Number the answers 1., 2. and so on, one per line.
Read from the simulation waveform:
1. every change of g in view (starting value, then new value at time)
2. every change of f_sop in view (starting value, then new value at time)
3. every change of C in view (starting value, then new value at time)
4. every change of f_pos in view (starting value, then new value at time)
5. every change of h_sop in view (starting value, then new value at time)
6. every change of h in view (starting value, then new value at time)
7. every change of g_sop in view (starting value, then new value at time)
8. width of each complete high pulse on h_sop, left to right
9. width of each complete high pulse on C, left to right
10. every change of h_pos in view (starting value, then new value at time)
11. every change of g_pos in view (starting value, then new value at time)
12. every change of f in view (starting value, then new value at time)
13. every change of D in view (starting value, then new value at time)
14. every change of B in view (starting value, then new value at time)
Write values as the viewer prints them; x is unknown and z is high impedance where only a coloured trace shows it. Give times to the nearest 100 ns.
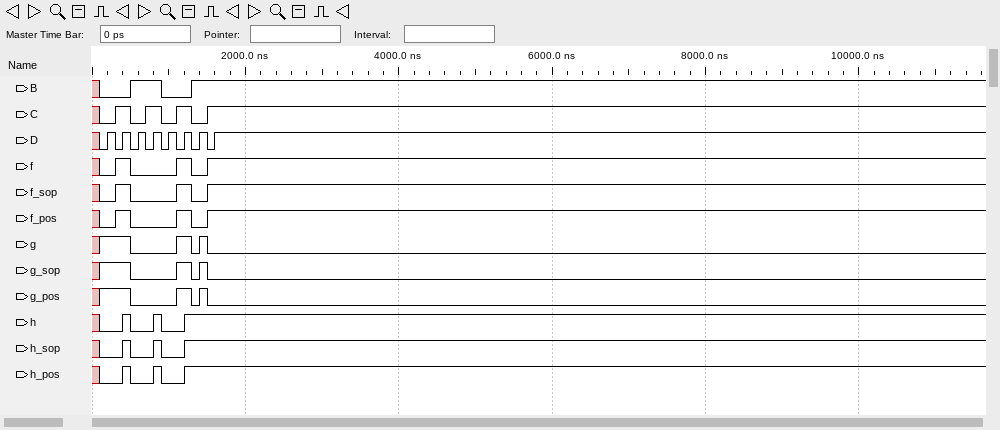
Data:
1. x, 1 at 100 ns, 0 at 500 ns, 1 at 1100 ns, 0 at 1300 ns, 1 at 1400 ns, 0 at 1500 ns
2. x, 0 at 100 ns, 1 at 300 ns, 0 at 500 ns, 1 at 1100 ns, 0 at 1300 ns, 1 at 1500 ns
3. x, 0 at 100 ns, 1 at 300 ns, 0 at 500 ns, 1 at 700 ns, 0 at 900 ns, 1 at 1100 ns, 0 at 1300 ns, 1 at 1500 ns
4. x, 0 at 100 ns, 1 at 300 ns, 0 at 500 ns, 1 at 1100 ns, 0 at 1300 ns, 1 at 1500 ns
5. x, 0 at 100 ns, 1 at 400 ns, 0 at 500 ns, 1 at 800 ns, 0 at 900 ns, 1 at 1200 ns
6. x, 0 at 100 ns, 1 at 400 ns, 0 at 500 ns, 1 at 800 ns, 0 at 900 ns, 1 at 1200 ns
7. x, 1 at 100 ns, 0 at 500 ns, 1 at 1100 ns, 0 at 1300 ns, 1 at 1400 ns, 0 at 1500 ns
8. 100 ns, 100 ns
9. 200 ns, 200 ns, 200 ns
10. x, 0 at 100 ns, 1 at 400 ns, 0 at 500 ns, 1 at 800 ns, 0 at 900 ns, 1 at 1200 ns
11. x, 1 at 100 ns, 0 at 500 ns, 1 at 1100 ns, 0 at 1300 ns, 1 at 1400 ns, 0 at 1500 ns
12. x, 0 at 100 ns, 1 at 300 ns, 0 at 500 ns, 1 at 1100 ns, 0 at 1300 ns, 1 at 1500 ns
13. x, 0 at 100 ns, 1 at 200 ns, 0 at 300 ns, 1 at 400 ns, 0 at 500 ns, 1 at 600 ns, 0 at 700 ns, 1 at 800 ns, 0 at 900 ns, 1 at 1000 ns, 0 at 1100 ns, 1 at 1200 ns, 0 at 1300 ns, 1 at 1400 ns, 0 at 1500 ns, 1 at 1600 ns
14. x, 0 at 100 ns, 1 at 500 ns, 0 at 900 ns, 1 at 1300 ns
